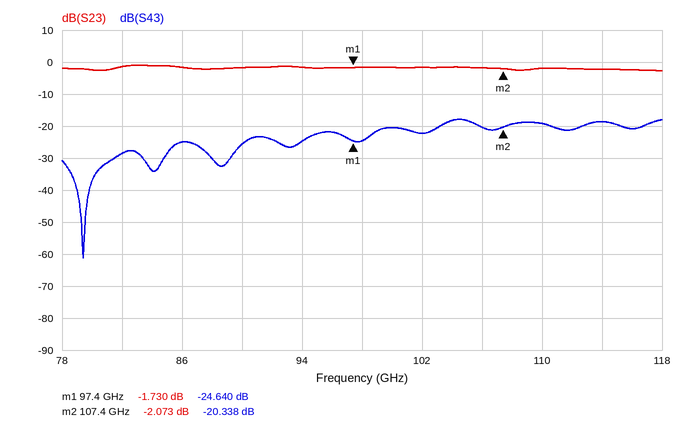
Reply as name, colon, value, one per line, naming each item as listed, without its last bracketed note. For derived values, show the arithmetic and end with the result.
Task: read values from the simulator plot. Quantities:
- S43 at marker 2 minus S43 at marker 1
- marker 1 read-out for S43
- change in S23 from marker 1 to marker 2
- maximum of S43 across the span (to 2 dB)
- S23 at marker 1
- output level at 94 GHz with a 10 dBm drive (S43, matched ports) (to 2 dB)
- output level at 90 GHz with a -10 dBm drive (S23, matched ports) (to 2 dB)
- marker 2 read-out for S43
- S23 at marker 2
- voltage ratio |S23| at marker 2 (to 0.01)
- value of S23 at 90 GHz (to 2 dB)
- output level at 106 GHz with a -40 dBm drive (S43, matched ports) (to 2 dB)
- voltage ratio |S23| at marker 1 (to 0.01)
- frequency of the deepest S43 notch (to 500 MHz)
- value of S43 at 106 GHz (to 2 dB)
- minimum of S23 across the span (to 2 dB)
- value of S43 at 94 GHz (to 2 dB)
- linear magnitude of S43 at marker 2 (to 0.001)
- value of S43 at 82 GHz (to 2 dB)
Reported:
S43 at marker 2 minus S43 at marker 1: -20.338 − (-24.64) = 4.302 dB
marker 1 read-out for S43: -24.640 dB
change in S23 from marker 1 to marker 2: -2.073 − (-1.73) = -0.343 dB
maximum of S43 across the span: -18 dB
S23 at marker 1: -1.730 dB
output level at 94 GHz with a 10 dBm drive (S43, matched ports): 10 dBm + (-24 dB) = -14 dBm
output level at 90 GHz with a -10 dBm drive (S23, matched ports): -10 dBm + (-2 dB) = -12 dBm
marker 2 read-out for S43: -20.338 dB
S23 at marker 2: -2.073 dB
voltage ratio |S23| at marker 2: 10^(-2.073/20) ≈ 0.79
value of S23 at 90 GHz: -2 dB
output level at 106 GHz with a -40 dBm drive (S43, matched ports): -40 dBm + (-20 dB) = -60 dBm
voltage ratio |S23| at marker 1: 10^(-1.73/20) ≈ 0.82
frequency of the deepest S43 notch: 79.5 GHz
value of S43 at 106 GHz: -20 dB
minimum of S23 across the span: -2 dB
value of S43 at 94 GHz: -24 dB
linear magnitude of S43 at marker 2: 10^(-20.338/20) ≈ 0.096
value of S43 at 82 GHz: -28 dB
